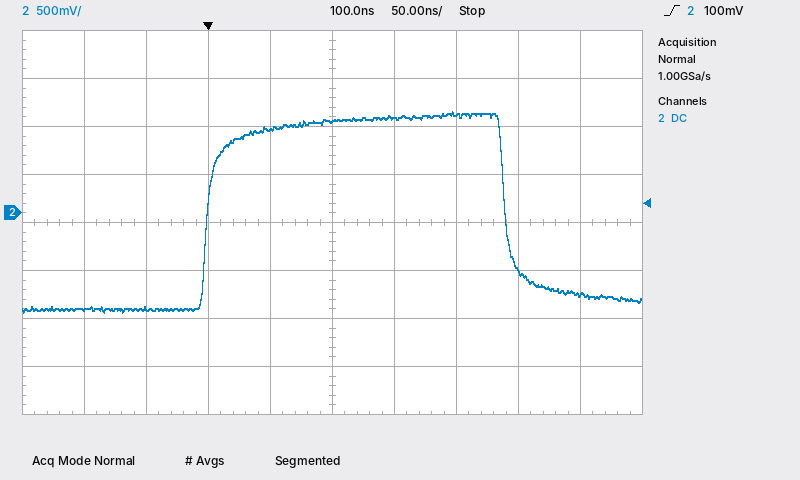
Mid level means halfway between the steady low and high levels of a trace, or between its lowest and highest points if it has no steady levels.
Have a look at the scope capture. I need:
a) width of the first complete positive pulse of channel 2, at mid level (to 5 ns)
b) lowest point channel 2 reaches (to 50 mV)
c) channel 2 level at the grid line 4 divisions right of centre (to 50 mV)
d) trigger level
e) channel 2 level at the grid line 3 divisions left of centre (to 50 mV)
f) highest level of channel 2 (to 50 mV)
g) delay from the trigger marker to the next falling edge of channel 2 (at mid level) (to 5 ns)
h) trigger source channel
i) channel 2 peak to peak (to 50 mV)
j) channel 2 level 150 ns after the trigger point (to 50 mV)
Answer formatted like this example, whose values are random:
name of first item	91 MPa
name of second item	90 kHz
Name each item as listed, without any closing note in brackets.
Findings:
width of the first complete positive pulse of channel 2, at mid level	240 ns
lowest point channel 2 reaches	-1.05 V
channel 2 level at the grid line 4 divisions right of centre	-850 mV
trigger level	100 mV
channel 2 level at the grid line 3 divisions left of centre	-1.00 V
highest level of channel 2	1.05 V
delay from the trigger marker to the next falling edge of channel 2 (at mid level)	240 ns
trigger source channel	channel 2
channel 2 peak to peak	2.10 V
channel 2 level 150 ns after the trigger point	1.00 V
